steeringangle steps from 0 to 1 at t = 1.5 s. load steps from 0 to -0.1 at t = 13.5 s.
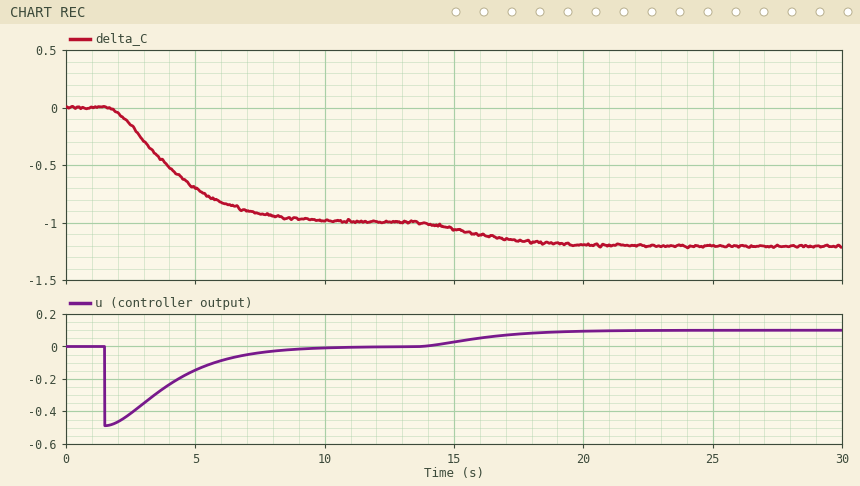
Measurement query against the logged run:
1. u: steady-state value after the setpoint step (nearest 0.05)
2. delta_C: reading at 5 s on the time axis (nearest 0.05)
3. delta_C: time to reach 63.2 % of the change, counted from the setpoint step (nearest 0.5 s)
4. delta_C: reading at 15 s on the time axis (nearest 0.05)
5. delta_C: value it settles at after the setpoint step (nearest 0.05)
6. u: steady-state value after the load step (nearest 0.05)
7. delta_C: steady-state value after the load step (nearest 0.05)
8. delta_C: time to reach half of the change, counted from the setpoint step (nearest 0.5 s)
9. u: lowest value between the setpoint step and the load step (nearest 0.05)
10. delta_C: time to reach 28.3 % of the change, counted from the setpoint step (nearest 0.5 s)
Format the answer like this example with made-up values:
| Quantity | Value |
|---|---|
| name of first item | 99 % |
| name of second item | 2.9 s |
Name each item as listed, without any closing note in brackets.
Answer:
| Quantity | Value |
|---|---|
| u: steady-state value after the setpoint step | 0.00 |
| delta_C: reading at 5 s on the time axis | -0.70 |
| delta_C: time to reach 63.2 % of the change, counted from the setpoint step | 3.0 s |
| delta_C: reading at 15 s on the time axis | -1.05 |
| delta_C: value it settles at after the setpoint step | -1.00 |
| u: steady-state value after the load step | 0.10 |
| delta_C: steady-state value after the load step | -1.20 |
| delta_C: time to reach half of the change, counted from the setpoint step | 2.5 s |
| u: lowest value between the setpoint step and the load step | -0.50 |
| delta_C: time to reach 28.3 % of the change, counted from the setpoint step | 1.5 s |
